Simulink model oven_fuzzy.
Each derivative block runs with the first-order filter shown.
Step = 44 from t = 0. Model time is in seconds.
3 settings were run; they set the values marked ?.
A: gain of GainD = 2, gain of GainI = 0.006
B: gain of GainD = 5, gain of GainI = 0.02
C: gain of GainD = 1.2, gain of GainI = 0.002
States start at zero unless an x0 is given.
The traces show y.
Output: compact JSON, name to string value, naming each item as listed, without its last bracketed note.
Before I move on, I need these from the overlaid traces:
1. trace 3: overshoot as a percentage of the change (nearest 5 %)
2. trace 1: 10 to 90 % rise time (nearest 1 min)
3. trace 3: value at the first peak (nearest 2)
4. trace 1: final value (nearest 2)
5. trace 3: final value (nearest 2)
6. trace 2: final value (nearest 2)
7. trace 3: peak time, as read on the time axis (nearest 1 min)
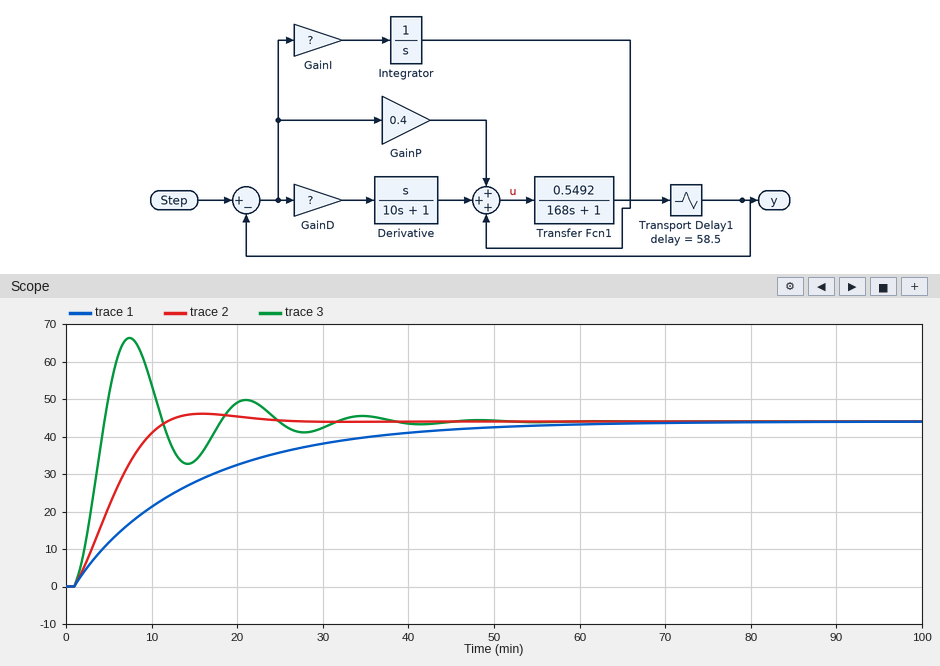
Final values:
{"trace 3: overshoot as a percentage of the change": "50 %", "trace 1: 10 to 90 % rise time": "32 min", "trace 3: value at the first peak": "66", "trace 1: final value": "44", "trace 3: final value": "44", "trace 2: final value": "44", "trace 3: peak time, as read on the time axis": "7 min"}
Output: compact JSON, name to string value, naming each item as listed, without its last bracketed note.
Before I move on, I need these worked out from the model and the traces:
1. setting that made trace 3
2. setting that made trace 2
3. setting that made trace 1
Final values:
{"setting that made trace 3": "B", "setting that made trace 2": "A", "setting that made trace 1": "C"}
